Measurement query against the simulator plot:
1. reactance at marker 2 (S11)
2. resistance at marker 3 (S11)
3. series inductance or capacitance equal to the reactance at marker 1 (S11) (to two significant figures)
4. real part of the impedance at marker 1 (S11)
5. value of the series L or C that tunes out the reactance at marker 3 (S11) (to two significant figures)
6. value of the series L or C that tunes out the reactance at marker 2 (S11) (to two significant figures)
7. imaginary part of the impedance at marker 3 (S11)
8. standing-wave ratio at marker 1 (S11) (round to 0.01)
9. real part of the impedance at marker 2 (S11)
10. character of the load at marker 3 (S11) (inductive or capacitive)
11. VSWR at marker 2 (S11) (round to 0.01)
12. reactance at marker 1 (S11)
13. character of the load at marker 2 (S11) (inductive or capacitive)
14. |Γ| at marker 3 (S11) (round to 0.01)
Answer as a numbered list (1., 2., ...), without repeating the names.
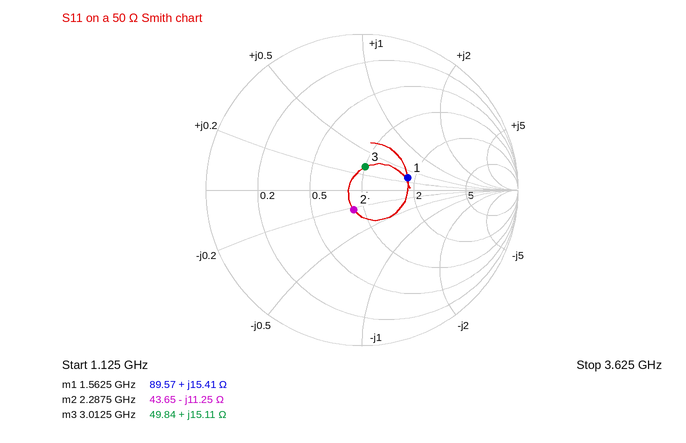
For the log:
1. -11.25 Ω
2. 49.84 Ω
3. 1.6 nH
4. 89.57 Ω
5. 3.5 pF
6. 780 pH
7. +15.11 Ω
8. 1.87
9. 43.65 Ω
10. inductive
11. 1.32
12. +15.41 Ω
13. capacitive
14. 0.15
